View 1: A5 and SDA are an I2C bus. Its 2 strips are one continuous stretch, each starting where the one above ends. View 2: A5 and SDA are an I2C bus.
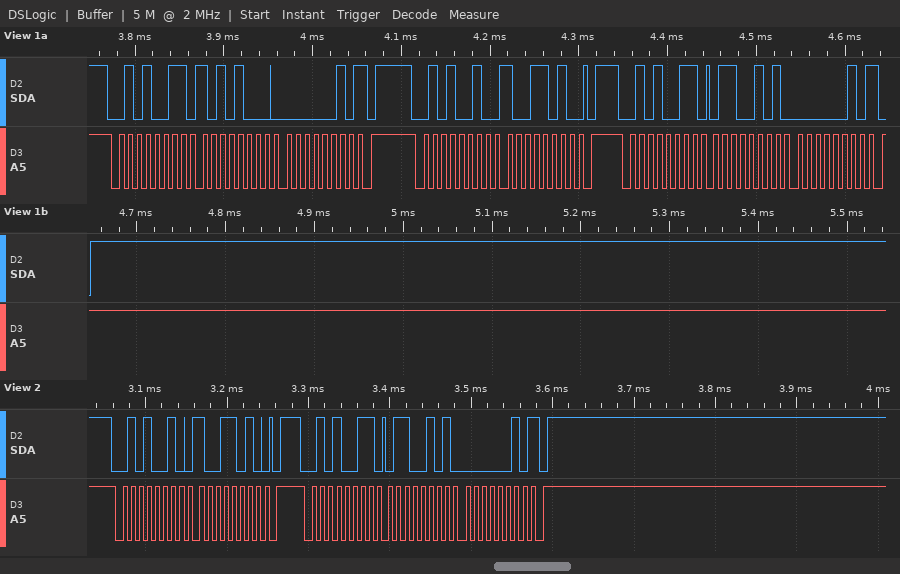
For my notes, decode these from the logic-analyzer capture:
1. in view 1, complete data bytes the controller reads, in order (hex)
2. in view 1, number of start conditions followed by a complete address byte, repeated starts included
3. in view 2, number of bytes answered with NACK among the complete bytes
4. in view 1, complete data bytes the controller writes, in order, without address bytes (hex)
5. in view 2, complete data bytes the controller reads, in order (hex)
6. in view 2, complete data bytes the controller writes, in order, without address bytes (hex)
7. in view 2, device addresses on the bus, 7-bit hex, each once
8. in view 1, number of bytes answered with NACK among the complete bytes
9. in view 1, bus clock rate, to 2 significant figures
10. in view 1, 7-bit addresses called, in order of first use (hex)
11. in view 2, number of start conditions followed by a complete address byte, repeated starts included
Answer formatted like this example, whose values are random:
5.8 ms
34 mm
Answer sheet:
A8 02 65 02
3
1
9A
65 02
9A
0x29
2
100 kHz
0x29
2
